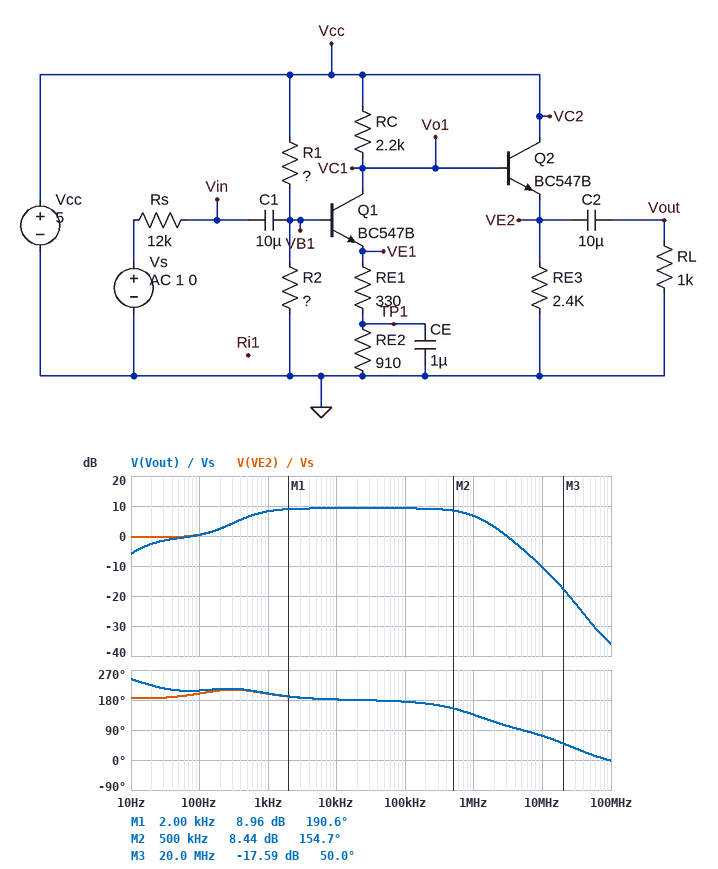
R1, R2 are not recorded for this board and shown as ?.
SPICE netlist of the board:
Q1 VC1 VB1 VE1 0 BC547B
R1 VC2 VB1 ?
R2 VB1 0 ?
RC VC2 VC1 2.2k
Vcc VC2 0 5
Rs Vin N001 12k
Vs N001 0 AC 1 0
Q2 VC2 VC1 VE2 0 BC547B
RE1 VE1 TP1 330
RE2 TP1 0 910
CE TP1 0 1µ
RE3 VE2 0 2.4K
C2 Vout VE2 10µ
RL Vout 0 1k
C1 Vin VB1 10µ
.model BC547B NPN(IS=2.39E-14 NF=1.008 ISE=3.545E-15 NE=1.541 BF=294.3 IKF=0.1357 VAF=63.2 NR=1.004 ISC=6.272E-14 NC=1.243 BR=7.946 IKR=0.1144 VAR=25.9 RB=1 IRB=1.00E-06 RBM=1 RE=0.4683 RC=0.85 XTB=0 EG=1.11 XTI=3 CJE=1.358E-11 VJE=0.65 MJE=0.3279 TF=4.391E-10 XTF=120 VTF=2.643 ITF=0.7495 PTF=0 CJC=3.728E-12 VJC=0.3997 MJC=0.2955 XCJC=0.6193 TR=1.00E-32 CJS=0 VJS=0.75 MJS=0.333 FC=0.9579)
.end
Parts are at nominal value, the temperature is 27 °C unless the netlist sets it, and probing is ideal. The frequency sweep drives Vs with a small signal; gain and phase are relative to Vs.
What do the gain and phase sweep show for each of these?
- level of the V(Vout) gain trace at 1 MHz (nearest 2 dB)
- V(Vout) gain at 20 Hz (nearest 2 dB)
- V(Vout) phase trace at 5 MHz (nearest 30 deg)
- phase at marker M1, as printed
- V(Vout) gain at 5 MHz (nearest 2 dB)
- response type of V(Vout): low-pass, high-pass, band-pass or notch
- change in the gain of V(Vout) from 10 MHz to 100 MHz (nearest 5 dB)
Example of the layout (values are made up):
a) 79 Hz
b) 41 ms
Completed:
a) 6 dB
b) -2 dB
c) 90 deg
d) 190.6 deg
e) -4 dB
f) band-pass
g) -25 dB
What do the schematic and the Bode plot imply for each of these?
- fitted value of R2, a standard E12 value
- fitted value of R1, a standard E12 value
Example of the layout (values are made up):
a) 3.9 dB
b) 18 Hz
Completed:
a) 22 kΩ
b) 82 kΩ
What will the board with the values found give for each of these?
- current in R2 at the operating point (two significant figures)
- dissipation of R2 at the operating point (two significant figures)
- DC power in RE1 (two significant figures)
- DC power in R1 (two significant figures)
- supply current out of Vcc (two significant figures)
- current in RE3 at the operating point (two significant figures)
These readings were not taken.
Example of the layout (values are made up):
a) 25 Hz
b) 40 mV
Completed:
a) 47 µA
b) 49 µW
c) 39 µW
d) 190 µW
e) 1.9 mA
f) 1.5 mA
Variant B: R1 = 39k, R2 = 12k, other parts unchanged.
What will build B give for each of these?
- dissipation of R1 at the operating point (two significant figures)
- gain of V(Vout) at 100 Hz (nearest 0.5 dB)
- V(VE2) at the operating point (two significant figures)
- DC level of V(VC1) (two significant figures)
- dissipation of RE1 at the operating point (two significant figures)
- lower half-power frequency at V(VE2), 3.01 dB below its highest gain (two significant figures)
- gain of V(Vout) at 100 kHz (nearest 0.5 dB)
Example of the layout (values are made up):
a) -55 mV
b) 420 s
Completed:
a) 380 µW
b) -2.0 dB
c) 3.4 V
d) 4.0 V
e) 64 µW
f) 510 Hz
g) 7.0 dB
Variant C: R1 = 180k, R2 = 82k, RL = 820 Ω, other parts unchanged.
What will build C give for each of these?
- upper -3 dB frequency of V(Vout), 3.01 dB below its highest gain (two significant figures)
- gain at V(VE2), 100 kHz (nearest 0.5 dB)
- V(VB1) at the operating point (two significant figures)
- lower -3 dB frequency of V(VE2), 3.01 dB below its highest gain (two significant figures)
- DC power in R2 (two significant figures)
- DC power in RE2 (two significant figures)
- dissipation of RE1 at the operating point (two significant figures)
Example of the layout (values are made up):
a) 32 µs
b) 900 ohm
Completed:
a) 810 kHz
b) 12.5 dB
c) 1.4 V
d) 510 Hz
e) 25 µW
f) 390 µW
g) 140 µW
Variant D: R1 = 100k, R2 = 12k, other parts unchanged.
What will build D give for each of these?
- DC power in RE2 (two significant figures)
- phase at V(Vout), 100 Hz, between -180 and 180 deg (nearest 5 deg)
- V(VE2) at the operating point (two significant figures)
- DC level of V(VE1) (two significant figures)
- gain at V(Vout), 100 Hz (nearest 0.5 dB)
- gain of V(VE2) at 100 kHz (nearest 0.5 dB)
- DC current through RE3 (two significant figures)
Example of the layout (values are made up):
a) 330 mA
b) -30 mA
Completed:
a) 130 nW
b) -165 deg
c) 4.3 V
d) 15 mV
e) -10.5 dB
f) -8.0 dB
g) 1.8 mA
